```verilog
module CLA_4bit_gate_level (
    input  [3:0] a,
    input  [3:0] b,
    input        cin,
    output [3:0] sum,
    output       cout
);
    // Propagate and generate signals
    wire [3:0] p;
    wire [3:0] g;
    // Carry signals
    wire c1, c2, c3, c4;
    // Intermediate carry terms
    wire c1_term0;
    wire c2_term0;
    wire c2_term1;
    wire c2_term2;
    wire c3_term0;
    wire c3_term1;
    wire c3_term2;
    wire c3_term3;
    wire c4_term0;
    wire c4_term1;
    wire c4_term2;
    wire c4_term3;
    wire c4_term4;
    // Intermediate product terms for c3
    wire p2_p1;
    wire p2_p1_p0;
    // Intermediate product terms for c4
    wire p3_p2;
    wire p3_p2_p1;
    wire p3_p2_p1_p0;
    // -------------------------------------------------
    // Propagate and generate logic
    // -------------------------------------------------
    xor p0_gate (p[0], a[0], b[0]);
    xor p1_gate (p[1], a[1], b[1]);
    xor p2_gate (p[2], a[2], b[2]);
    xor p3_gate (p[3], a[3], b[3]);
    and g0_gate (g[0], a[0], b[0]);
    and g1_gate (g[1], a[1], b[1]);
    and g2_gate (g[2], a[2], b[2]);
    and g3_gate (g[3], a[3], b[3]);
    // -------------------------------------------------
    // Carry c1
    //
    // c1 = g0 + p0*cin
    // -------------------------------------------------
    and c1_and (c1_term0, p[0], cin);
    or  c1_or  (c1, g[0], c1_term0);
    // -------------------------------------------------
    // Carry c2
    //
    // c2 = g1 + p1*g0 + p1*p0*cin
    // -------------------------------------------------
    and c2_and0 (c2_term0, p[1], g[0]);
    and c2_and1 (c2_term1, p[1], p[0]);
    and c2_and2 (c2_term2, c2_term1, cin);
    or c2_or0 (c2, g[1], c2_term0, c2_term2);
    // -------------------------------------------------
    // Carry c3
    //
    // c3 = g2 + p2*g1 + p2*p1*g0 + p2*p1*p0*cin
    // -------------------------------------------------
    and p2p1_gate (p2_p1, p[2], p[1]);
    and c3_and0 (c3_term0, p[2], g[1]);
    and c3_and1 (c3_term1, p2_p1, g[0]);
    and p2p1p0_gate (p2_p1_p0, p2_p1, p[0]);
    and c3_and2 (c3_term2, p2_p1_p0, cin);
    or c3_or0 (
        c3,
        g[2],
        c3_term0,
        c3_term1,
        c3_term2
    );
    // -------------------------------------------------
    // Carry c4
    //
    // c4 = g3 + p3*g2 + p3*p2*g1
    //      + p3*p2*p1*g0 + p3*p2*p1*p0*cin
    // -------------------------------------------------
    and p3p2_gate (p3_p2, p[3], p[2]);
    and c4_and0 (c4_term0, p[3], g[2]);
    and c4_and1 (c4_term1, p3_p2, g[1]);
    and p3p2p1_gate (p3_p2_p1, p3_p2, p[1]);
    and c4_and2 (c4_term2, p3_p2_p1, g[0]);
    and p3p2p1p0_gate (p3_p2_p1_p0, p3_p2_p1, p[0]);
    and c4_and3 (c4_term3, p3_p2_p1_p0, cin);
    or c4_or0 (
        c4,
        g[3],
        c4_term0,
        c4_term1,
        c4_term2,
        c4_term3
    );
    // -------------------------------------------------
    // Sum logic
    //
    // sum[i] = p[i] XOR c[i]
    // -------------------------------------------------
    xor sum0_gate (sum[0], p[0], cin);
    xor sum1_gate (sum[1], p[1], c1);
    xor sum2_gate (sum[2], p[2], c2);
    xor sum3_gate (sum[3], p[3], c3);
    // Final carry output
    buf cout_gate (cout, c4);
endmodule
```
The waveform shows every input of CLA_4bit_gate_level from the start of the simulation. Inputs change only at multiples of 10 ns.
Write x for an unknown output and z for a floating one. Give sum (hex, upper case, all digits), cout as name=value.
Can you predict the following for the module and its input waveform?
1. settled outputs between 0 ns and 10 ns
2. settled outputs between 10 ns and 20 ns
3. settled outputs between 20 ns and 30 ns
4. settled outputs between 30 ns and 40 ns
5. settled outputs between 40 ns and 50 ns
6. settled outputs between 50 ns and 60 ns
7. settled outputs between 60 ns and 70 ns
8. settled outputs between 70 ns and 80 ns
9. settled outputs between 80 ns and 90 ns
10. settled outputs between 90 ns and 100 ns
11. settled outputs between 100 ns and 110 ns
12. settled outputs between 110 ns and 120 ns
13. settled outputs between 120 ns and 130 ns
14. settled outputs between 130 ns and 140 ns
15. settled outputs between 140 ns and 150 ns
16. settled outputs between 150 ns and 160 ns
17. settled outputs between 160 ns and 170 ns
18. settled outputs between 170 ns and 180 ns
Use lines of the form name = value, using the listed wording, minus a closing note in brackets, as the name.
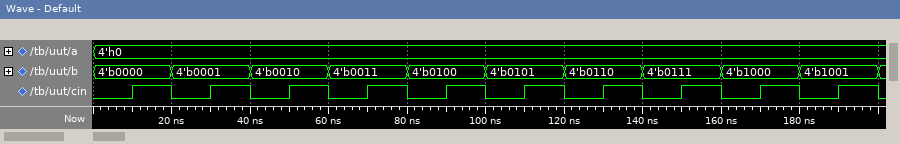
settled outputs between 0 ns and 10 ns = sum=0, cout=0
settled outputs between 10 ns and 20 ns = sum=1, cout=0
settled outputs between 20 ns and 30 ns = sum=1, cout=0
settled outputs between 30 ns and 40 ns = sum=2, cout=0
settled outputs between 40 ns and 50 ns = sum=2, cout=0
settled outputs between 50 ns and 60 ns = sum=3, cout=0
settled outputs between 60 ns and 70 ns = sum=3, cout=0
settled outputs between 70 ns and 80 ns = sum=4, cout=0
settled outputs between 80 ns and 90 ns = sum=4, cout=0
settled outputs between 90 ns and 100 ns = sum=5, cout=0
settled outputs between 100 ns and 110 ns = sum=5, cout=0
settled outputs between 110 ns and 120 ns = sum=6, cout=0
settled outputs between 120 ns and 130 ns = sum=6, cout=0
settled outputs between 130 ns and 140 ns = sum=7, cout=0
settled outputs between 140 ns and 150 ns = sum=7, cout=0
settled outputs between 150 ns and 160 ns = sum=8, cout=0
settled outputs between 160 ns and 170 ns = sum=8, cout=0
settled outputs between 170 ns and 180 ns = sum=9, cout=0
